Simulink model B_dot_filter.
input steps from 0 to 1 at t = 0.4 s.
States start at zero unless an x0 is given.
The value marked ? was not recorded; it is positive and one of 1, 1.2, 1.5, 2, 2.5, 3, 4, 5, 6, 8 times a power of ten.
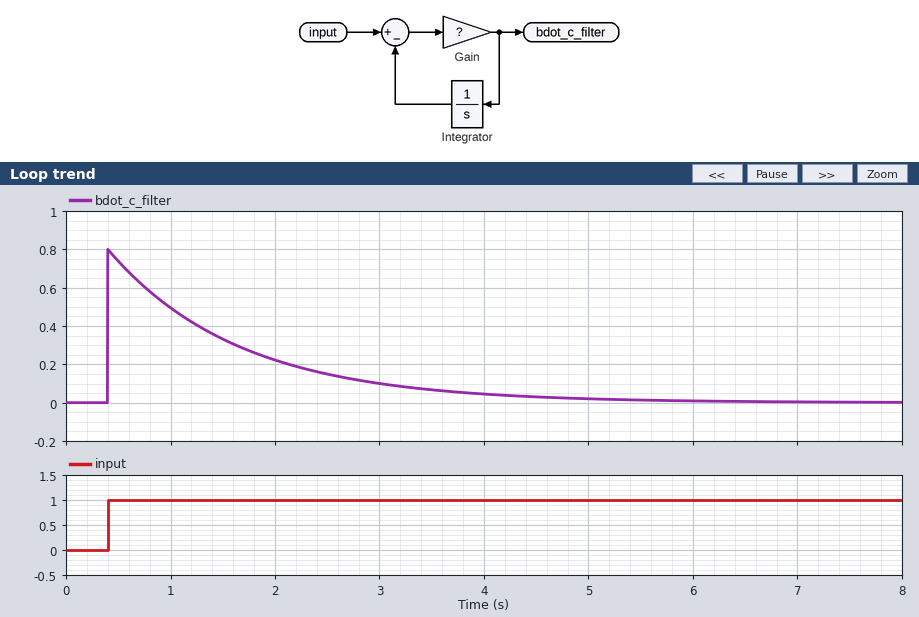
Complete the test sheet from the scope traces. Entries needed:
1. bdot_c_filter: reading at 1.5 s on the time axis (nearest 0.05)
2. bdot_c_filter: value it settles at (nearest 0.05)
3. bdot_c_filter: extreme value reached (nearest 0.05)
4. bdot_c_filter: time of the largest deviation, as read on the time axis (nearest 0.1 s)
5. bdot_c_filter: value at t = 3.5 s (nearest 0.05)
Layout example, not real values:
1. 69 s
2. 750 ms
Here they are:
1. 0.35
2. 0.00
3. 0.80
4. 0.4 s
5. 0.05
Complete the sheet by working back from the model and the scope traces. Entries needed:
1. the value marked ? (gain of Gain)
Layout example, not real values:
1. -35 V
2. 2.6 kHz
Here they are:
1. 0.8
